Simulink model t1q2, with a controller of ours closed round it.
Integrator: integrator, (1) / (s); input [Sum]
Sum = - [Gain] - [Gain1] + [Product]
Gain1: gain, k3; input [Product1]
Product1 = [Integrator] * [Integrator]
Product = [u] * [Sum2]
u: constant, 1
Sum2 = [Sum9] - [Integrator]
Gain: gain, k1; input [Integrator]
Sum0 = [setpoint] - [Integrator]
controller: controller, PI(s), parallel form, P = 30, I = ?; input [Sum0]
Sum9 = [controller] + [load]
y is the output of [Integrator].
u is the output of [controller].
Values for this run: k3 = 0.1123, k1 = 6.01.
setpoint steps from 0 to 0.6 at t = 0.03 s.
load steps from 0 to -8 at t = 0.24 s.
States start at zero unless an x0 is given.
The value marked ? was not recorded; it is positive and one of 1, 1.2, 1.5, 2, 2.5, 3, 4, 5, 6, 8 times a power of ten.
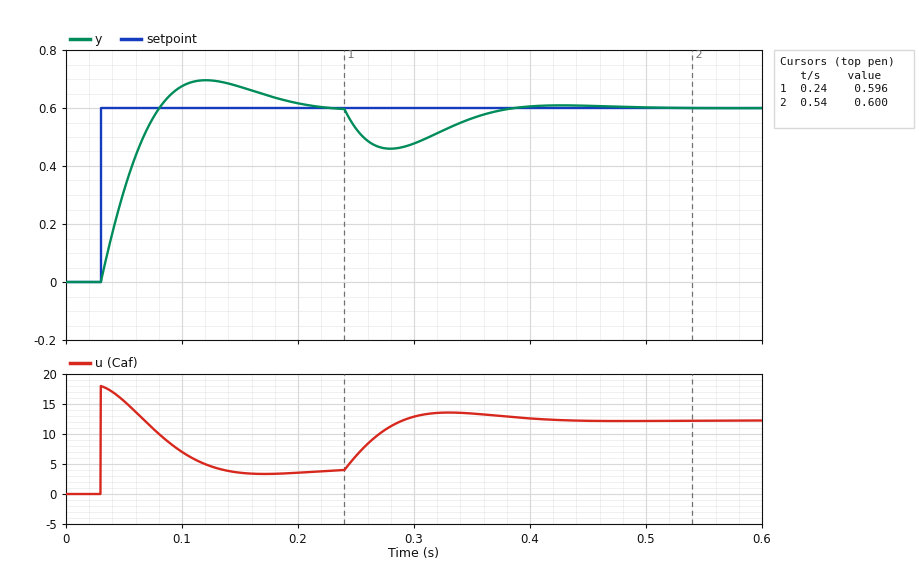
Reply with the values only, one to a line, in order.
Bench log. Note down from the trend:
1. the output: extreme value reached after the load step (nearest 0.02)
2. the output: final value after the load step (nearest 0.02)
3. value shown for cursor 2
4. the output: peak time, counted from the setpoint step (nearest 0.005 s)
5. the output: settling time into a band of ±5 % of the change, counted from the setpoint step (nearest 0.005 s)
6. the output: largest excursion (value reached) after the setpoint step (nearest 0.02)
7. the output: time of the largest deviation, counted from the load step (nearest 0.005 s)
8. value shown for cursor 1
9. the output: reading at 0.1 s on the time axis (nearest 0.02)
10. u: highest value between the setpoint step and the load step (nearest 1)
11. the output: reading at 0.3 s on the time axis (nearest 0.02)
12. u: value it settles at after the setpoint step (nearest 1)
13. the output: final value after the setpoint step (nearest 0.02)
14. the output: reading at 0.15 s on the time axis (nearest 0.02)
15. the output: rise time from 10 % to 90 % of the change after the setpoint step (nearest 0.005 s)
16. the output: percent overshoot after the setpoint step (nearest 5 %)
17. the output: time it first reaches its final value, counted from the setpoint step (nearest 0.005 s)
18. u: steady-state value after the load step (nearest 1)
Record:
0.46
0.60
0.600
0.090 s
0.155 s
0.70
0.040 s
0.596
0.68
18
0.48
4
0.60
0.68
0.040 s
15 %
0.050 s
12
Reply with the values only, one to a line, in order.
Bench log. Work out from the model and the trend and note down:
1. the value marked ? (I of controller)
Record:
800
